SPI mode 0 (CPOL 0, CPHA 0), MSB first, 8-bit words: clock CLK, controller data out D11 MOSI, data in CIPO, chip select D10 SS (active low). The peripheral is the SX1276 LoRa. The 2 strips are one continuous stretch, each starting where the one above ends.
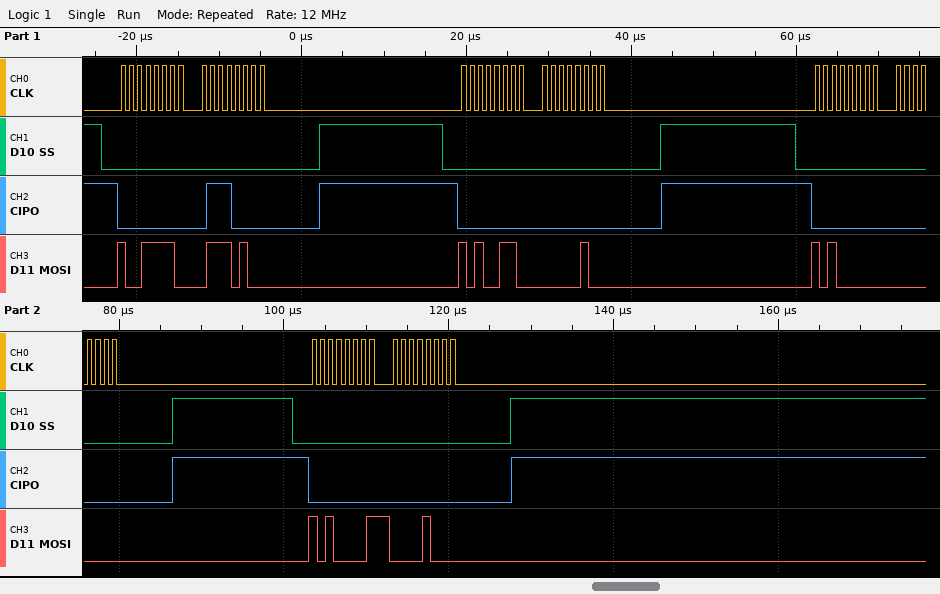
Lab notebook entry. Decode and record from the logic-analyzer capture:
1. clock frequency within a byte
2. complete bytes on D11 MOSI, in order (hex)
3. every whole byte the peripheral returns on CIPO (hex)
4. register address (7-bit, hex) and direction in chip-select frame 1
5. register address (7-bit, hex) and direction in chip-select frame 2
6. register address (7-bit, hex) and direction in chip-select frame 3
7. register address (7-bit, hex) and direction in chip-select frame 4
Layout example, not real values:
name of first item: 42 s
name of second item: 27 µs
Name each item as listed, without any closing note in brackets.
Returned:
clock frequency within a byte: 1 MHz
complete bytes on D11 MOSI, in order: 0x9E 0x74 0xA6 0x04 0xA0 0x00 0xA1 0x08
every whole byte the peripheral returns on CIPO: 0x00 0x70 0x00 0x00 0x00 0x00 0x00 0x00
register address (7-bit, hex) and direction in chip-select frame 1: 0x1E write
register address (7-bit, hex) and direction in chip-select frame 2: 0x26 write
register address (7-bit, hex) and direction in chip-select frame 3: 0x20 write
register address (7-bit, hex) and direction in chip-select frame 4: 0x21 write
